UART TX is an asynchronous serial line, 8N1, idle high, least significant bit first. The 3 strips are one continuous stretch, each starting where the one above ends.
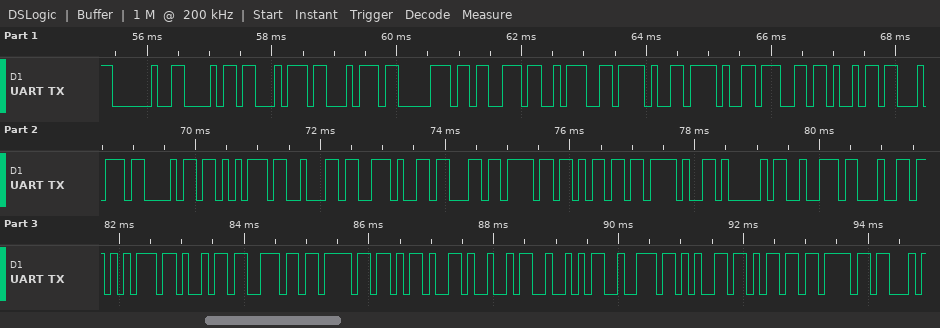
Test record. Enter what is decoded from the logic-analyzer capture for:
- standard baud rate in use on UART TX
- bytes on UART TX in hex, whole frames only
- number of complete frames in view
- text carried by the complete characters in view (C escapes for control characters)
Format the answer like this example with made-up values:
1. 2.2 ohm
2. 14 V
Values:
1. 9600 baud
2. 0x20 0x68 0x74 0x74 0x70 0x73 0x3A 0x2F 0x2F 0x67 0x69 0x74 0x68 0x75 0x62 0x2E 0x63 0x6F 0x6D 0x2F 0x41 0x72 0x64 0x75 0x69 0x6E 0x6F 0x2D 0x49 0x52 0x72 0x65 0x6D 0x6F
3. 34
4. " https://github.com/Arduino-IRremo"
